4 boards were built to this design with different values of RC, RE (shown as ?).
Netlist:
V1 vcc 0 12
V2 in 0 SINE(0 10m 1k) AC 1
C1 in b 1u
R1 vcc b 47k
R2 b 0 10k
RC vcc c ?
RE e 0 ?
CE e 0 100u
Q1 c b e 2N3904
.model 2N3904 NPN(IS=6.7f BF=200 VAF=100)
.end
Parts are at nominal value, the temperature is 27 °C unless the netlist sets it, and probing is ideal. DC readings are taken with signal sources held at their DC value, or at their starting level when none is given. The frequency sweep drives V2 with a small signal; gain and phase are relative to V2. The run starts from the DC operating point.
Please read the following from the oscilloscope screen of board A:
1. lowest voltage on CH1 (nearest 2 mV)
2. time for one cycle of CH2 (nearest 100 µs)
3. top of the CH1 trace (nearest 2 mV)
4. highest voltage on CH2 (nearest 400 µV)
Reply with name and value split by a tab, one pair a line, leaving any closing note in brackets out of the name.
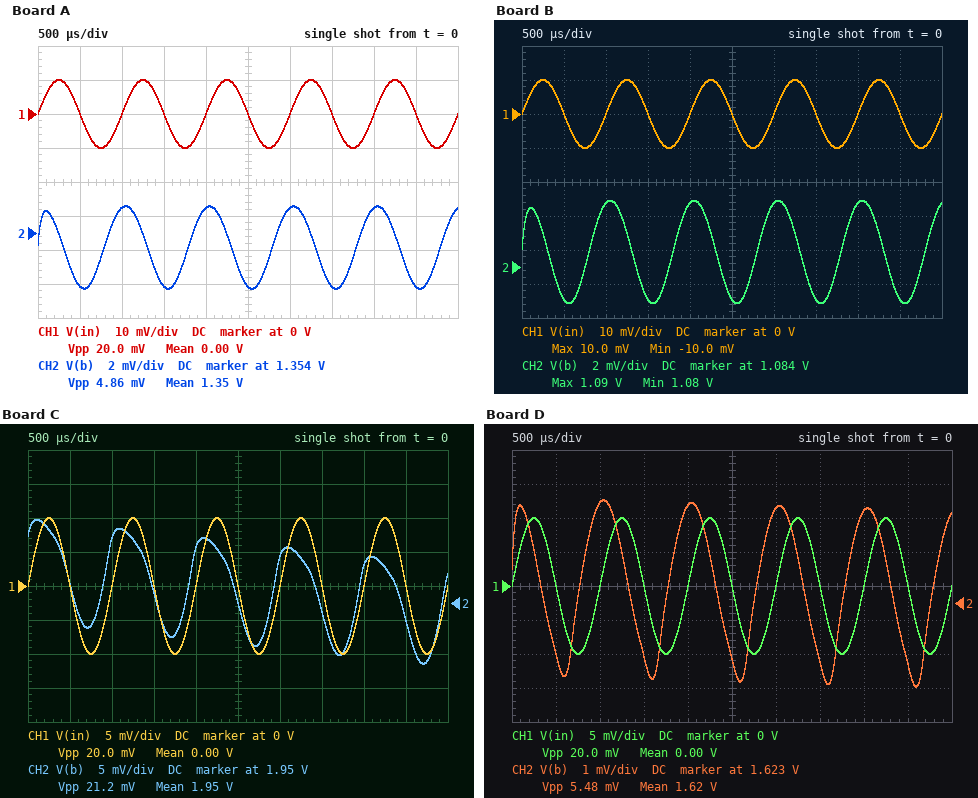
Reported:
lowest voltage on CH1	-10 mV
time for one cycle of CH2	1.0 ms
top of the CH1 trace	10 mV
highest voltage on CH2	1.3556 V
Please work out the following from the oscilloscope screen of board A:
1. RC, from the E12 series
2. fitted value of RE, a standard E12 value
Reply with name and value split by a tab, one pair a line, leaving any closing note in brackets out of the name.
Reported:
RC, from the E12 series	10 kΩ
fitted value of RE, a standard E12 value	560 Ω
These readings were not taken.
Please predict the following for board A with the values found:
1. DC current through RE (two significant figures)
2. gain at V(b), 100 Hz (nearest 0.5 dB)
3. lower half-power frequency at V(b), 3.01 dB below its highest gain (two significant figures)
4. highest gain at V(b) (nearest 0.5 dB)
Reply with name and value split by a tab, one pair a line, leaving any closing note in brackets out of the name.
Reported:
DC current through RE	1.2 mA
gain at V(b), 100 Hz	-31.5 dB
lower half-power frequency at V(b), 3.01 dB below its highest gain	4.0 kHz
highest gain at V(b)	0 dB
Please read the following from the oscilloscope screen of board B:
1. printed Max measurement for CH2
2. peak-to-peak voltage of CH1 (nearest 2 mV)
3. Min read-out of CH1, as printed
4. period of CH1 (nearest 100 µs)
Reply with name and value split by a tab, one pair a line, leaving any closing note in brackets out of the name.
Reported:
printed Max measurement for CH2	1.09 V
peak-to-peak voltage of CH1	20 mV
Min read-out of CH1, as printed	-10.0 mV
period of CH1	1.0 ms
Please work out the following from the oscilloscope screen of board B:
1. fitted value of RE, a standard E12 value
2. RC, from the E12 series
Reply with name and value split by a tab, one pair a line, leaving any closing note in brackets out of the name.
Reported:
fitted value of RE, a standard E12 value	470 Ω
RC, from the E12 series	15 kΩ
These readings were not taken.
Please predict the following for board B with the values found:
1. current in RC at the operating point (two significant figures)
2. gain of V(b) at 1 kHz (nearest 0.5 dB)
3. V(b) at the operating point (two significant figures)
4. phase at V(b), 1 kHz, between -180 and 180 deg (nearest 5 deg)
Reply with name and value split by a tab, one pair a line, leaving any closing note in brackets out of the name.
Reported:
current in RC at the operating point	770 µA
gain of V(b) at 1 kHz	-10.5 dB
V(b) at the operating point	1.1 V
phase at V(b), 1 kHz, between -180 and 180 deg	70 deg
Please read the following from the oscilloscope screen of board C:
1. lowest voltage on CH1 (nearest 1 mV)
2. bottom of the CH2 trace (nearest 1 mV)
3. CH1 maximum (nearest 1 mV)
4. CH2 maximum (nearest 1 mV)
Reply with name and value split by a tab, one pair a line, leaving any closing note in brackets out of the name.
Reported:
lowest voltage on CH1	-10 mV
bottom of the CH2 trace	1.941 V
CH1 maximum	10 mV
CH2 maximum	1.962 V
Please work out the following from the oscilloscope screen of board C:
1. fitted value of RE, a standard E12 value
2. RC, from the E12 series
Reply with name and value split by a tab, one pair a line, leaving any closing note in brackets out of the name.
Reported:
fitted value of RE, a standard E12 value	1.2 kΩ
RC, from the E12 series	10 kΩ
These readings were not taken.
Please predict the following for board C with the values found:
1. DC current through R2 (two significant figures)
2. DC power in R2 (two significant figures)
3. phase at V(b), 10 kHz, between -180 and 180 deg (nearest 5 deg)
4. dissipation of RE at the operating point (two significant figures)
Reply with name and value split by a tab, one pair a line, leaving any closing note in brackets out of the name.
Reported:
DC current through R2	200 µA
DC power in R2	380 µW
phase at V(b), 10 kHz, between -180 and 180 deg	15 deg
dissipation of RE at the operating point	1.4 mW
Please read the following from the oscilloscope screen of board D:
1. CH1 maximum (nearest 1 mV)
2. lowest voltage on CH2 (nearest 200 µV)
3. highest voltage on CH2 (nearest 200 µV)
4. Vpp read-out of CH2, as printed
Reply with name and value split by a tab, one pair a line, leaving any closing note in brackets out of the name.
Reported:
CH1 maximum	10 mV
lowest voltage on CH2	1.6206 V
highest voltage on CH2	1.6260 V
Vpp read-out of CH2, as printed	5.48 mV
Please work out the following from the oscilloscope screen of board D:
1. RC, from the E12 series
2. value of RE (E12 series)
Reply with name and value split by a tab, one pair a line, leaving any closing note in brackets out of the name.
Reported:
RC, from the E12 series	8.2 kΩ
value of RE	680 Ω
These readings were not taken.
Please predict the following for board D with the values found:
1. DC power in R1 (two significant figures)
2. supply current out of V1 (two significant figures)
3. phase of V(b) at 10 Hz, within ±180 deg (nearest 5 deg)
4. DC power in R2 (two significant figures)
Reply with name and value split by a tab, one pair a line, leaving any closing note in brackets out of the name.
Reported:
DC power in R1	2.3 mW
supply current out of V1	1.6 mA
phase of V(b) at 10 Hz, within ±180 deg	25 deg
DC power in R2	260 µW
